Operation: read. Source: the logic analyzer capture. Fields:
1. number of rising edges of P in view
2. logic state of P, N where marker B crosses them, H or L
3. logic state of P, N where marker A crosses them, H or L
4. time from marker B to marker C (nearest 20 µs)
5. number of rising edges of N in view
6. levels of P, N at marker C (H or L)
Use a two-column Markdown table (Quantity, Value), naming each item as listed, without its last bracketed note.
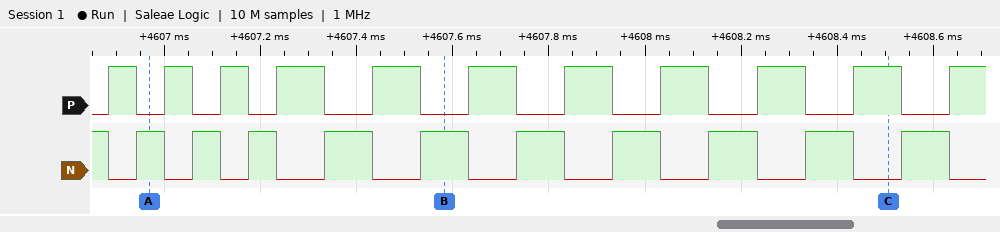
| Quantity | Value |
|---|---|
| number of rising edges of P in view | 11 |
| logic state of P, N where marker B crosses them, H or L | P=L, N=H |
| logic state of P, N where marker A crosses them, H or L | P=L, N=H |
| time from marker B to marker C | 920 µs |
| number of rising edges of N in view | 10 |
| levels of P, N at marker C | P=H, N=L |
